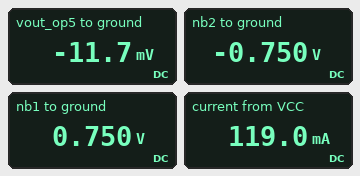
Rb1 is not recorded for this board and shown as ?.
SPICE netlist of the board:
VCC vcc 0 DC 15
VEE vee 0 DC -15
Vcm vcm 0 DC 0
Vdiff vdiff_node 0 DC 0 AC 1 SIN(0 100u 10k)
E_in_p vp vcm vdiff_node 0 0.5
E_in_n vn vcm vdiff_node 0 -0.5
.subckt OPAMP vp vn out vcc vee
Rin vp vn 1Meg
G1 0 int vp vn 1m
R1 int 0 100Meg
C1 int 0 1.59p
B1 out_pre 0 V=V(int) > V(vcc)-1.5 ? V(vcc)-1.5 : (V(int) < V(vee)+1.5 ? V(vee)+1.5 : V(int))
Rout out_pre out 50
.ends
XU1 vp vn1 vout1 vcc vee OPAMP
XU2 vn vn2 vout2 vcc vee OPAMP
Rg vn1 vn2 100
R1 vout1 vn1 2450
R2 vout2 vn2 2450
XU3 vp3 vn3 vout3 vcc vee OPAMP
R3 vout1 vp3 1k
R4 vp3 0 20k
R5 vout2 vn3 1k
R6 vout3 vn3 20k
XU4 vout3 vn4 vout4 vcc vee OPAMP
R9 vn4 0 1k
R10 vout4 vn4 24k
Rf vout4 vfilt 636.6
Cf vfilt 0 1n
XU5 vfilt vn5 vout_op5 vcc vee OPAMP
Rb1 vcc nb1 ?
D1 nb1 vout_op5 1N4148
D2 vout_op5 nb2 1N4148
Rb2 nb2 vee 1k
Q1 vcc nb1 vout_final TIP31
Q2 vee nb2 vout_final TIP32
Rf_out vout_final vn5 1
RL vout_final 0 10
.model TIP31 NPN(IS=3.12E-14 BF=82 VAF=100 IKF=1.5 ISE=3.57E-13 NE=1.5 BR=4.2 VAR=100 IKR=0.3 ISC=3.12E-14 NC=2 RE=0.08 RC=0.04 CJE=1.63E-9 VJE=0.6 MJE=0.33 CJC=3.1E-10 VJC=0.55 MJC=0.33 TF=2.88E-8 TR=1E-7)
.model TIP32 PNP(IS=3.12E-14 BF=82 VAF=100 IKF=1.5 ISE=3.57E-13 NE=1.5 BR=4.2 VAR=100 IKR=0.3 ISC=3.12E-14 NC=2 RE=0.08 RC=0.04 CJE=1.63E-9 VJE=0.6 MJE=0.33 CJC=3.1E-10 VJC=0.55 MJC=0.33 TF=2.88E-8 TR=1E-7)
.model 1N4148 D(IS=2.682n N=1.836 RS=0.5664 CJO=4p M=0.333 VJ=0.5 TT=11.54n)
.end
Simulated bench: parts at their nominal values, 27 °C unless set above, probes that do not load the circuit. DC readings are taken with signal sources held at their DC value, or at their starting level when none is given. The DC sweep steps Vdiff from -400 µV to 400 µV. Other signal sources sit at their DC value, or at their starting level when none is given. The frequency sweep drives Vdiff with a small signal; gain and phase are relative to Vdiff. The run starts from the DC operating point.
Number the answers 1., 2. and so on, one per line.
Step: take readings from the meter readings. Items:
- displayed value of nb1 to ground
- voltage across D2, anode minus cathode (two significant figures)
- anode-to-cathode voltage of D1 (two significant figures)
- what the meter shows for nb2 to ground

1. 0.750 V
2. 740 mV
3. 760 mV
4. -0.750 V
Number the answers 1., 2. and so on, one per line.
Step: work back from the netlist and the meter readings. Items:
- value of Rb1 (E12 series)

1. 680 Ω
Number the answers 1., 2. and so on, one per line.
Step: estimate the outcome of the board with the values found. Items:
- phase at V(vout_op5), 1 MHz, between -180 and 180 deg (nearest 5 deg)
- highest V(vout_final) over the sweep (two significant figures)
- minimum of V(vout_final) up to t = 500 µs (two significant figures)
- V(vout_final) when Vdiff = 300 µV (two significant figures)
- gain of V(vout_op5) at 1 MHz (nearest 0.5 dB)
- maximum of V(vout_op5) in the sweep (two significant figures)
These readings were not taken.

1. -130 deg
2. 6.7 V
3. -2.5 V
4. 6.7 V
5. 74.5 dB
6. 12 V
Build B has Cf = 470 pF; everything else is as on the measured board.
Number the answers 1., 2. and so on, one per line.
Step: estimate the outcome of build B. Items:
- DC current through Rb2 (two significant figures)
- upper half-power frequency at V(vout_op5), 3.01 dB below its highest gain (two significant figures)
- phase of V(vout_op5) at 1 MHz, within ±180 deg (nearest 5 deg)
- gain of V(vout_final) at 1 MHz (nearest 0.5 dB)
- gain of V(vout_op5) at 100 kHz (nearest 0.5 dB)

1. 14 mA
2. 490 kHz
3. -115 deg
4. 80.0 dB
5. 88.0 dB
